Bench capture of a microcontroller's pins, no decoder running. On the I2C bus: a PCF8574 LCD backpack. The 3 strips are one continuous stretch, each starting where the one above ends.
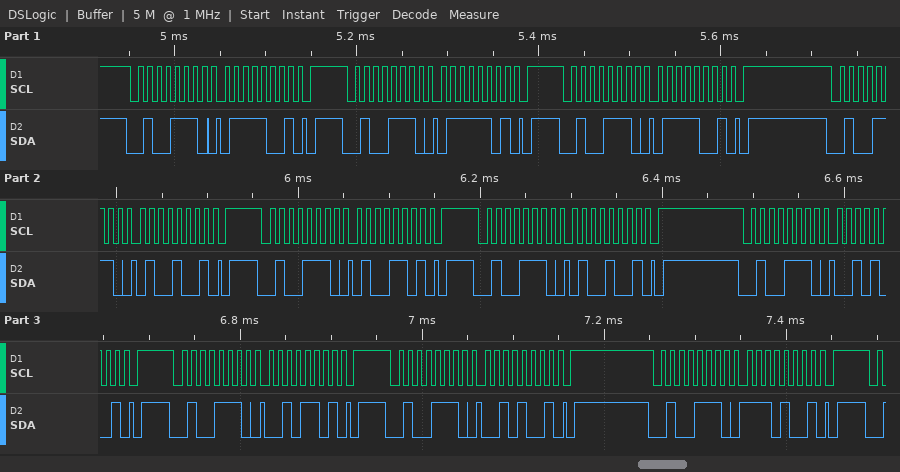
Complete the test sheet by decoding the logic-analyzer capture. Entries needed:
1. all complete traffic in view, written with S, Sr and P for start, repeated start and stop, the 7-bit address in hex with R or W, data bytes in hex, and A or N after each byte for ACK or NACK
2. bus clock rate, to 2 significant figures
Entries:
S 27W A 79 A P S 27W A 7D A P S 27W A 79 A P S 27W A 49 A P S 27W A 4D A P S 27W A 49 A P S 27W A 29 A P S 27W A 2D A P S 27W A 29 A P S 27W A E9 A P
100 kHz
